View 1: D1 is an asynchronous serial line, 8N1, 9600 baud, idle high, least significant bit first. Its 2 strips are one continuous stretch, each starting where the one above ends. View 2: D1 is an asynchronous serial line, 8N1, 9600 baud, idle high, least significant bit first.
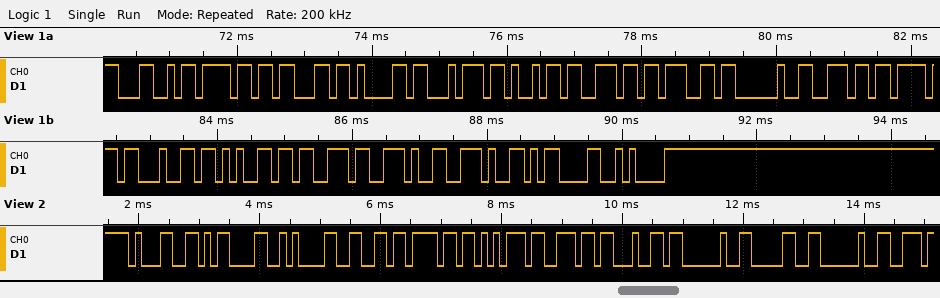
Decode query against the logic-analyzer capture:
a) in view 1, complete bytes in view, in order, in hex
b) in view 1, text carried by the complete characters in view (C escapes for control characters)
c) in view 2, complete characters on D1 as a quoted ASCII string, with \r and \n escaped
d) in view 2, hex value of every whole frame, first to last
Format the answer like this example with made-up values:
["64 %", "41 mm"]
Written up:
["0x4C 0x6F 0x63 0x61 0x74 0x69 0x6E 0x67 0x20 0x6E 0x6F 0x64 0x65 0x73 0x2E 0x2E 0x0D 0x0A", "\"Locating nodes..\\r\\n\"", "\"1\\r\\nfound 0 \"", "31 0D 0A 66 6F 75 6E 64 20 30 20"]
